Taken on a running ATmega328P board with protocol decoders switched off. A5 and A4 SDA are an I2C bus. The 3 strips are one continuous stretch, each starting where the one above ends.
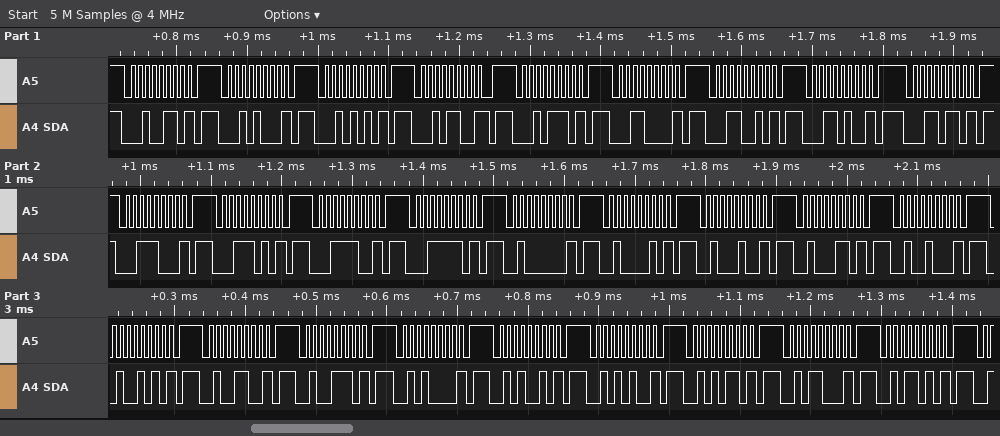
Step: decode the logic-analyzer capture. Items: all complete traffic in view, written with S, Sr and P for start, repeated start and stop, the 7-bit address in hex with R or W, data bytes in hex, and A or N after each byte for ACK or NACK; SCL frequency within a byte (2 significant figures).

S 13W N P S 14W N P S 15W N P S 16W N P S 17W N P S 18W N P S 19W N P S 1AW N P S 1BW N P S 1CW N P S 1DW N P S 1EW N P S 1FW N P S 20W N P S 21W N P S 22W N P S 23W N P S 24W N P S 25W N P S 26W N P S 27W N P S 28W N P S 29W N P S 2AW N P S 2BW N P S 2CW N P S 2DW N P
100 kHz
